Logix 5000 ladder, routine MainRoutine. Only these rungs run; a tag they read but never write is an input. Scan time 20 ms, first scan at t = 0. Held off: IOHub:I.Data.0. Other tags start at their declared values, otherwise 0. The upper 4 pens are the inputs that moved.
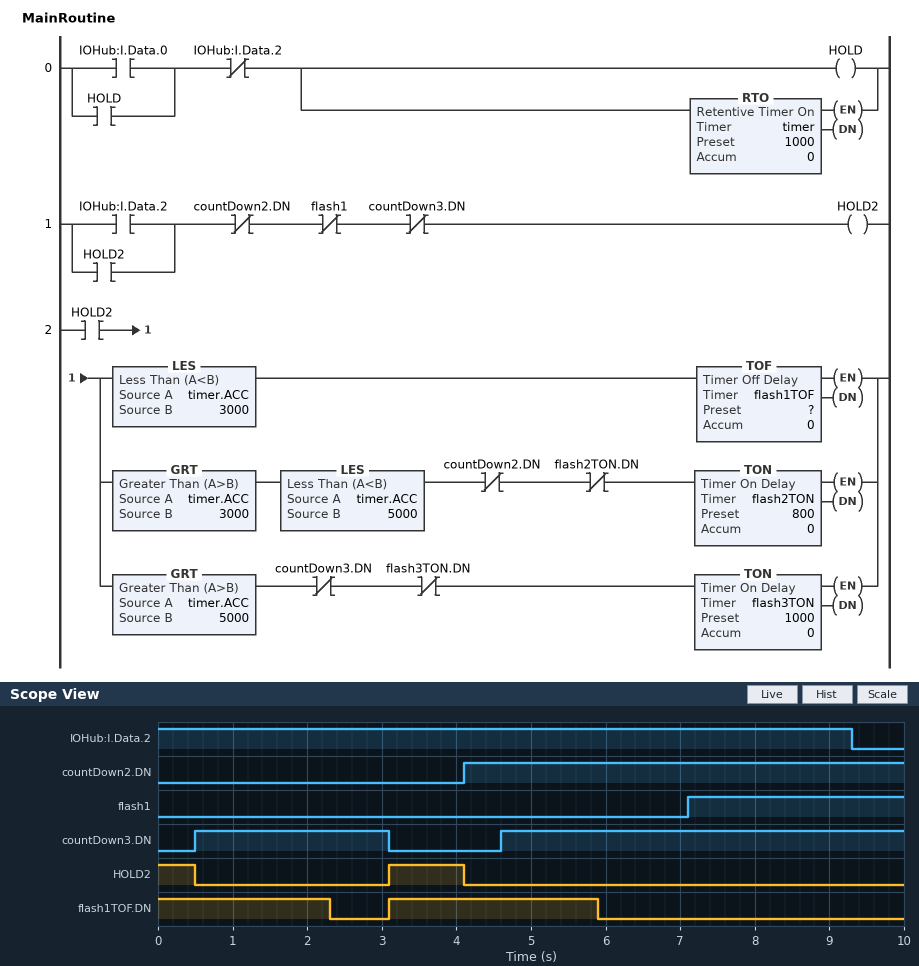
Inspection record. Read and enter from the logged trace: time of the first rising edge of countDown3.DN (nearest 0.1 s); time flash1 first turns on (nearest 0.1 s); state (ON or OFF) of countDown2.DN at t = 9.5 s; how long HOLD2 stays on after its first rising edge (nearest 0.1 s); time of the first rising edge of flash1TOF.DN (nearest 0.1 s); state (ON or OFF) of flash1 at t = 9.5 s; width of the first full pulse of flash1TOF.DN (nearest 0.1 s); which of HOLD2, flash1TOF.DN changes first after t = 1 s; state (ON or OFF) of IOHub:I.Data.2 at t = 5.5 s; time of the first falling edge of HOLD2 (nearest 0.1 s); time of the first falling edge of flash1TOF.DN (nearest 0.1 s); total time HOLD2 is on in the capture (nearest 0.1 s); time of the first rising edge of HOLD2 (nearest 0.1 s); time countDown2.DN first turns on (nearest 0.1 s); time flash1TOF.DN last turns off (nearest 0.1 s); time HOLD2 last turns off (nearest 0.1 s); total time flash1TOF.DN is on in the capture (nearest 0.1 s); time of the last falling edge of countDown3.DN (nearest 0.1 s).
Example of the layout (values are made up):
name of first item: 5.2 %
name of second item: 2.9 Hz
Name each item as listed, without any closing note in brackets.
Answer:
time of the first rising edge of countDown3.DN: 0.5 s
time flash1 first turns on: 7.1 s
state (ON or OFF) of countDown2.DN at t = 9.5 s: ON
how long HOLD2 stays on after its first rising edge: 1.0 s
time of the first rising edge of flash1TOF.DN: 3.1 s
state (ON or OFF) of flash1 at t = 9.5 s: ON
width of the first full pulse of flash1TOF.DN: 2.8 s
which of HOLD2, flash1TOF.DN changes first after t = 1 s: flash1TOF.DN
state (ON or OFF) of IOHub:I.Data.2 at t = 5.5 s: ON
time of the first falling edge of HOLD2: 0.5 s
time of the first falling edge of flash1TOF.DN: 2.3 s
total time HOLD2 is on in the capture: 1.5 s
time of the first rising edge of HOLD2: 3.1 s
time countDown2.DN first turns on: 4.1 s
time flash1TOF.DN last turns off: 5.9 s
time HOLD2 last turns off: 4.1 s
total time flash1TOF.DN is on in the capture: 5.1 s
time of the last falling edge of countDown3.DN: 3.1 s
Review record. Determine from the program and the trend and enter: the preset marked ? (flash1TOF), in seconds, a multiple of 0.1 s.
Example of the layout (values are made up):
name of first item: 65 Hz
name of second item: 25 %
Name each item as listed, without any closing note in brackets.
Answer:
the preset marked ? (flash1TOF), in seconds, a multiple of 0.1 s: 1.8 s
